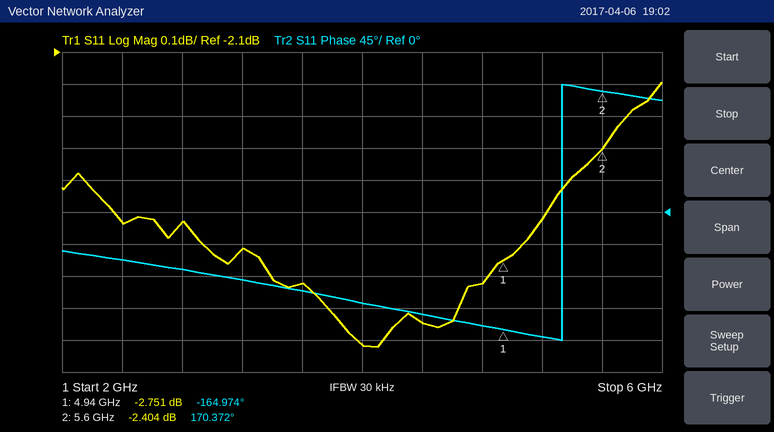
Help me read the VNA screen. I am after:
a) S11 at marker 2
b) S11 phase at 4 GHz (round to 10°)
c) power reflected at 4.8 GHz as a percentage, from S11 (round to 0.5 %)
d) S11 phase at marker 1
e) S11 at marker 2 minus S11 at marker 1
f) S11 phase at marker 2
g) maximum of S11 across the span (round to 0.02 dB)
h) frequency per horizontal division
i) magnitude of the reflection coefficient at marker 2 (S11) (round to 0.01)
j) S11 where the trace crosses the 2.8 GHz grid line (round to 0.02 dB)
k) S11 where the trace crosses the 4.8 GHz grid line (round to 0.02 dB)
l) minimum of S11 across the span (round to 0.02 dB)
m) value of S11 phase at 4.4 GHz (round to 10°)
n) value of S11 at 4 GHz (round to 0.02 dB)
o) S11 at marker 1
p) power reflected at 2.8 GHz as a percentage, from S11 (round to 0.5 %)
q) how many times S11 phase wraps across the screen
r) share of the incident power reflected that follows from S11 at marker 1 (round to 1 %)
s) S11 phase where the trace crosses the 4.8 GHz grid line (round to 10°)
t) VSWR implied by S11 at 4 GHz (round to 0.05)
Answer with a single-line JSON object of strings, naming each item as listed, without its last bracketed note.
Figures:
{"S11 at marker 2": "-2.404 dB", "S11 phase at 4 GHz": "-130°", "power reflected at 4.8 GHz as a percentage, from S11": "52.0 %", "S11 phase at marker 1": "-164.974°", "S11 at marker 2 minus S11 at marker 1": "0.347 dB", "S11 phase at marker 2": "170.372°", "maximum of S11 across the span": "-2.20 dB", "frequency per horizontal division": "400 MHz", "magnitude of the reflection coefficient at marker 2 (S11)": "0.76", "S11 where the trace crosses the 2.8 GHz grid line": "-2.64 dB", "S11 where the trace crosses the 4.8 GHz grid line": "-2.82 dB", "minimum of S11 across the span": "-3.02 dB", "value of S11 phase at 4.4 GHz": "-140°", "value of S11 at 4 GHz": "-3.02 dB", "S11 at marker 1": "-2.751 dB", "power reflected at 2.8 GHz as a percentage, from S11": "54.5 %", "how many times S11 phase wraps across the screen": "1", "share of the incident power reflected that follows from S11 at marker 1": "53 %", "S11 phase where the trace crosses the 4.8 GHz grid line": "-160°", "VSWR implied by S11 at 4 GHz": "5.80"}
